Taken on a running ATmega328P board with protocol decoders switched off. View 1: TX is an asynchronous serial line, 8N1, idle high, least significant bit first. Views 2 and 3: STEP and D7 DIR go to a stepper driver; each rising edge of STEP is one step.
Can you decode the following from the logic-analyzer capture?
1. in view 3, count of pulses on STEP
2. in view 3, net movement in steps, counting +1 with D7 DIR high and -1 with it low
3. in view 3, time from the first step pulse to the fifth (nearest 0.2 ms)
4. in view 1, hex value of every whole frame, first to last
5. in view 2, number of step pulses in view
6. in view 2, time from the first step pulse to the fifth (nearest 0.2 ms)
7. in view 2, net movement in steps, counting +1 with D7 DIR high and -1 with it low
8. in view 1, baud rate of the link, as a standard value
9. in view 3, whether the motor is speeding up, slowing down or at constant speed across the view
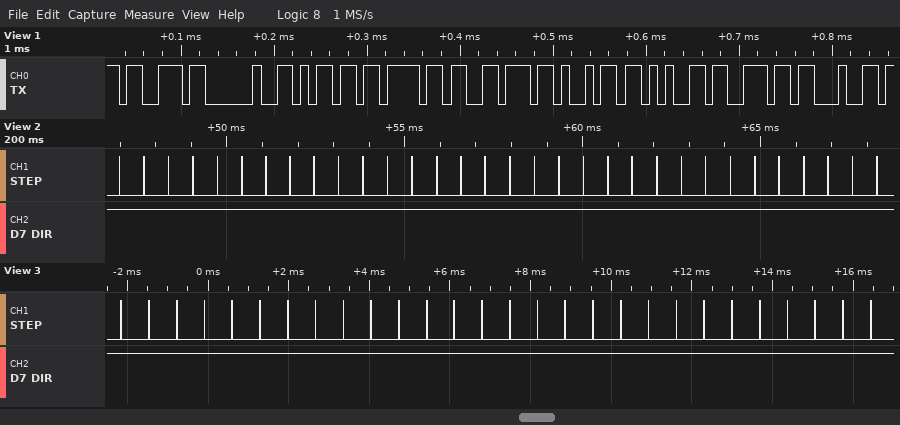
28
+28
2.8 ms
73 20 6D 6F 76 69 65 6E 64
32
2.8 ms
+32
115200 baud
constant speed
